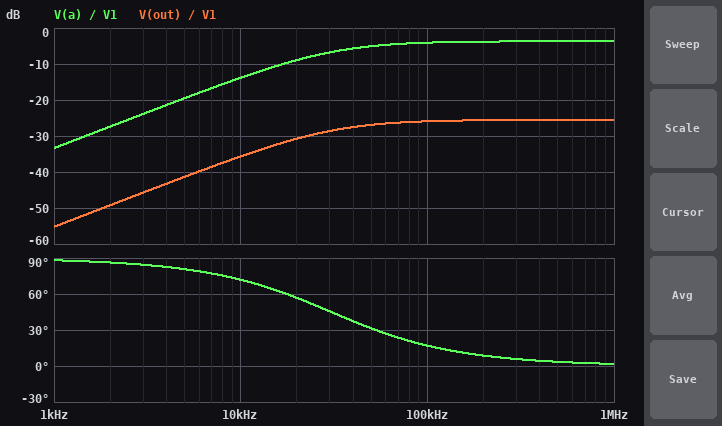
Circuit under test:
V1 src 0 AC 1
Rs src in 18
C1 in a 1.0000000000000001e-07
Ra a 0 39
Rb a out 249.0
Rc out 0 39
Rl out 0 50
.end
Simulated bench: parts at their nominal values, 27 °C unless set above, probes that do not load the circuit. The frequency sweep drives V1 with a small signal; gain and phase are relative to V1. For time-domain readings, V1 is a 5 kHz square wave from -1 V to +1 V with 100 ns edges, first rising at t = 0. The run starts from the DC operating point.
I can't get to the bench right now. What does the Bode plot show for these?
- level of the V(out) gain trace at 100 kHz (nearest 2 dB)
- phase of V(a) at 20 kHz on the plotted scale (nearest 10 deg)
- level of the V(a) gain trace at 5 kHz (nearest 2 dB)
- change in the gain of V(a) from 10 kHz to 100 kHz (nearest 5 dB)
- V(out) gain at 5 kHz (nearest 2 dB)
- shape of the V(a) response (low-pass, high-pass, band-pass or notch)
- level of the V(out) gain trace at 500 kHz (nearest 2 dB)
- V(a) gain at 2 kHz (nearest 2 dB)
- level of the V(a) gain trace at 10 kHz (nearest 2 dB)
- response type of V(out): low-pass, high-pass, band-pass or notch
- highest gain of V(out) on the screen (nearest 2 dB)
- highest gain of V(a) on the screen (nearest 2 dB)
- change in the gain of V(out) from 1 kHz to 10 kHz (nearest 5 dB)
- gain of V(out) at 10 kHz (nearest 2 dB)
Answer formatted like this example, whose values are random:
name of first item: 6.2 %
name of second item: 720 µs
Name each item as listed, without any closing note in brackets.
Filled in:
level of the V(out) gain trace at 100 kHz: -26 dB
phase of V(a) at 20 kHz on the plotted scale: 60 deg
level of the V(a) gain trace at 5 kHz: -20 dB
change in the gain of V(a) from 10 kHz to 100 kHz: 10 dB
V(out) gain at 5 kHz: -42 dB
shape of the V(a) response: high-pass
level of the V(out) gain trace at 500 kHz: -26 dB
V(a) gain at 2 kHz: -28 dB
level of the V(a) gain trace at 10 kHz: -14 dB
response type of V(out): low-pass, high-pass, band-pass or notch: high-pass
highest gain of V(out) on the screen: -26 dB
highest gain of V(a) on the screen: -4 dB
change in the gain of V(out) from 1 kHz to 10 kHz: 20 dB
gain of V(out) at 10 kHz: -36 dB
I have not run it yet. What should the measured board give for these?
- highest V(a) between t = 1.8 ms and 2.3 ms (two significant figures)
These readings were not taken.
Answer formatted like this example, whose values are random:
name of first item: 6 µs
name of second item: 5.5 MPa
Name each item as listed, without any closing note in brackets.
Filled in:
highest V(a) between t = 1.8 ms and 2.3 ms: 1.3 V
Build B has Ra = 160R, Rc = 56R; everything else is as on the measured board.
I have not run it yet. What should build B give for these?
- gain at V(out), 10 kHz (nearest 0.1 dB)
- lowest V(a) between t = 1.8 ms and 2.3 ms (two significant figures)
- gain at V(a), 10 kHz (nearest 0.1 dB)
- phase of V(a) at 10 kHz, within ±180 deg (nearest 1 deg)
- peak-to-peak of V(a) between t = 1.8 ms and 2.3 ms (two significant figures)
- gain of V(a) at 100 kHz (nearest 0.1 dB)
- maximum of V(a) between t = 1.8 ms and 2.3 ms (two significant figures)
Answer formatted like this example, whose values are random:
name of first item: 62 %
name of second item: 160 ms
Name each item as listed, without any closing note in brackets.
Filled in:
gain at V(out), 10 kHz: -26.2 dB
lowest V(a) between t = 1.8 ms and 2.3 ms: -1.7 V
gain at V(a), 10 kHz: -5.9 dB
phase of V(a) at 10 kHz, within ±180 deg: 53 deg
peak-to-peak of V(a) between t = 1.8 ms and 2.3 ms: 3.4 V
gain of V(a) at 100 kHz: -1.5 dB
maximum of V(a) between t = 1.8 ms and 2.3 ms: 1.7 V
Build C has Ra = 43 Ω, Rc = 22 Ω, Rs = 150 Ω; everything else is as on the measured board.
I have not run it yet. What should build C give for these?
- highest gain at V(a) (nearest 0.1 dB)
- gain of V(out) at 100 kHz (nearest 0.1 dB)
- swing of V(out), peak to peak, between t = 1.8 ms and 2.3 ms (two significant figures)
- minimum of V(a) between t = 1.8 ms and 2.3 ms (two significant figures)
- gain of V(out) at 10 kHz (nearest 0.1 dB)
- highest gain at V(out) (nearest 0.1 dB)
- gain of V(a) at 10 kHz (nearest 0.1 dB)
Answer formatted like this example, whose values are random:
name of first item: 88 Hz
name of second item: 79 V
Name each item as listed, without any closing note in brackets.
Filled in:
highest gain at V(a): -14.1 dB
gain of V(out) at 100 kHz: -38.9 dB
swing of V(out), peak to peak, between t = 1.8 ms and 2.3 ms: 45 mV
minimum of V(a) between t = 1.8 ms and 2.3 ms: -390 mV
gain of V(out) at 10 kHz: -41.2 dB
highest gain at V(out): -38.8 dB
gain of V(a) at 10 kHz: -16.4 dB
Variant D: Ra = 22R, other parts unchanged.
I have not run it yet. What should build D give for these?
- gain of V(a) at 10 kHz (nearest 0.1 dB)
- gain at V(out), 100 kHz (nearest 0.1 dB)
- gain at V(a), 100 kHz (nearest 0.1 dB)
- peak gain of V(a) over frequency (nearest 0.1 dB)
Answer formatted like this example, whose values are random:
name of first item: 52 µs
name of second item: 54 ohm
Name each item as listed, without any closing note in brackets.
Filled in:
gain of V(a) at 10 kHz: -18.1 dB
gain at V(out), 100 kHz: -28.0 dB
gain at V(a), 100 kHz: -6.2 dB
peak gain of V(a) over frequency: -5.5 dB
